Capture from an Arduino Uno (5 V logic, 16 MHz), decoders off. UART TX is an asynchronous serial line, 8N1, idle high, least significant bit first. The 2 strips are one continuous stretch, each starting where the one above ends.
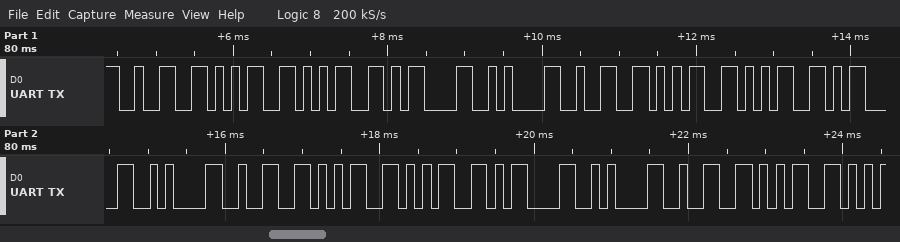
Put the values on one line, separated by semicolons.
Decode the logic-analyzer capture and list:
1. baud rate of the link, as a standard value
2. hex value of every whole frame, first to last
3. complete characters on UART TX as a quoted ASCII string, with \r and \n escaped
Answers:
9600 baud; 0x32 0x35 0x35 0x0D 0x0A 0x32 0x35 0x35 0x0D 0x0A 0x32 0x35 0x35 0x0D 0x0A 0x32 0x35; "255\r\n255\r\n255\r\n25"
